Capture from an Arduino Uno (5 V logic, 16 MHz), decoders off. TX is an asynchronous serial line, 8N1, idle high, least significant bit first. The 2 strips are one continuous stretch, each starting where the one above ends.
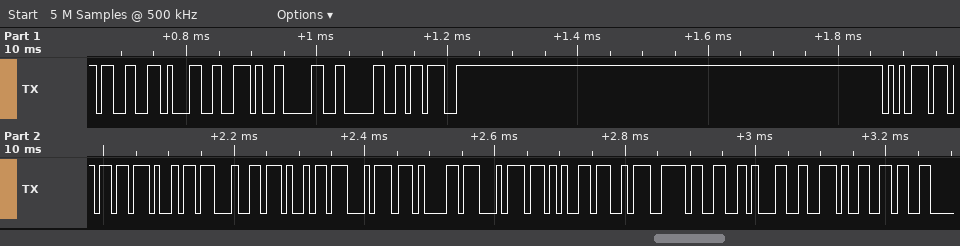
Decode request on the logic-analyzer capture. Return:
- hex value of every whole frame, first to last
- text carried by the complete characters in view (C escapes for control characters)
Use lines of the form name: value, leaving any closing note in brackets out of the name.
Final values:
hex value of every whole frame, first to last: 33 31 2E 30 30 3B 75 6D 69 64 69 74 61 74 65 3A 33 31 2E 36
text carried by the complete characters in view: "31.00;umiditate:31.6"
